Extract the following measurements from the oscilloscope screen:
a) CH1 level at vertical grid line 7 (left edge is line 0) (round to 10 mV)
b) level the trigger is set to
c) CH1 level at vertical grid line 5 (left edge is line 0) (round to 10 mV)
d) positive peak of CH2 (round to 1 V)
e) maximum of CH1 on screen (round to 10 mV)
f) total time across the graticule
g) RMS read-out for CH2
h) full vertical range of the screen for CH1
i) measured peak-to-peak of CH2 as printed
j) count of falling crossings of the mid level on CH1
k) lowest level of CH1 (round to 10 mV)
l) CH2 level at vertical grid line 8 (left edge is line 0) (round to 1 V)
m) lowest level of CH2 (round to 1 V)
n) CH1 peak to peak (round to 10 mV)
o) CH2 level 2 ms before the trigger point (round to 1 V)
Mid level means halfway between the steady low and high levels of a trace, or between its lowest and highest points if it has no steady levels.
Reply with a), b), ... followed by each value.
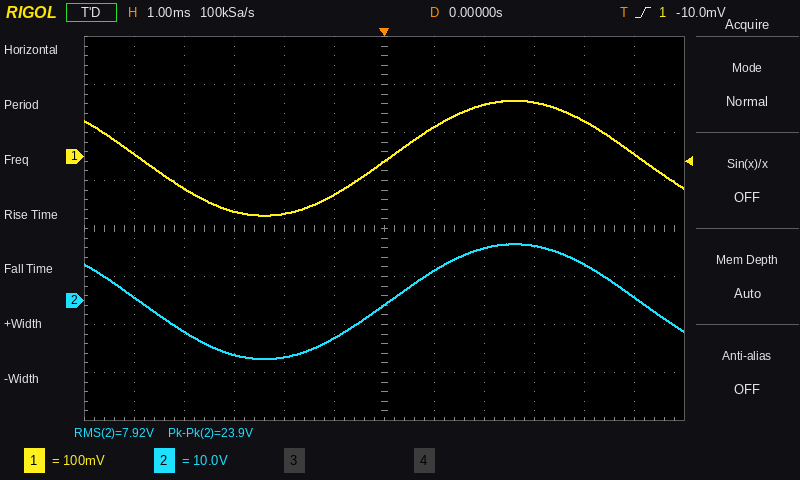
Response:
a) 60 mV
b) -10.0 mV
c) -80 mV
d) 12 V
e) 120 mV
f) 12 ms
g) 7.92 V
h) 800 mV
i) 23.9 V
j) 2
k) -120 mV
l) 11 V
m) -12 V
n) 240 mV
o) -12 V
